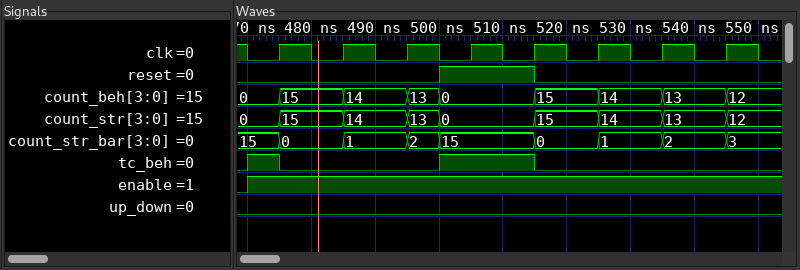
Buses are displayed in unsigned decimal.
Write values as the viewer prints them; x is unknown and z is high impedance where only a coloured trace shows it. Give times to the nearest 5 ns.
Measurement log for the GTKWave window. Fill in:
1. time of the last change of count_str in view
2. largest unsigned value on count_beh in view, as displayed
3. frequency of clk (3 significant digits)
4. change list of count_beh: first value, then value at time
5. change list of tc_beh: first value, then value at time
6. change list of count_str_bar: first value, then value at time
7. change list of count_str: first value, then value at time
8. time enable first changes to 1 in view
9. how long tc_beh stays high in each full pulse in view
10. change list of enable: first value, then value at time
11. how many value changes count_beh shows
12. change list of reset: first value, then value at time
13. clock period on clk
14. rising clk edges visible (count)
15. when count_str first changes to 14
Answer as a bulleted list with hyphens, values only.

- 545 ns
- 15
- 100 MHz
- 0, 15 at 475 ns, 14 at 485 ns, 13 at 495 ns, 0 at 500 ns, 15 at 515 ns, 14 at 525 ns, 13 at 535 ns, 12 at 545 ns
- 0, 1 at 470 ns, 0 at 475 ns, 1 at 500 ns, 0 at 515 ns
- 15, 0 at 475 ns, 1 at 485 ns, 2 at 495 ns, 15 at 500 ns, 0 at 515 ns, 1 at 525 ns, 2 at 535 ns, 3 at 545 ns
- 0, 15 at 475 ns, 14 at 485 ns, 13 at 495 ns, 0 at 500 ns, 15 at 515 ns, 14 at 525 ns, 13 at 535 ns, 12 at 545 ns
- 470 ns
- 5 ns, 15 ns
- 0, 1 at 470 ns
- 8
- 0, 1 at 500 ns, 0 at 515 ns
- 10 ns
- 8
- 485 ns
